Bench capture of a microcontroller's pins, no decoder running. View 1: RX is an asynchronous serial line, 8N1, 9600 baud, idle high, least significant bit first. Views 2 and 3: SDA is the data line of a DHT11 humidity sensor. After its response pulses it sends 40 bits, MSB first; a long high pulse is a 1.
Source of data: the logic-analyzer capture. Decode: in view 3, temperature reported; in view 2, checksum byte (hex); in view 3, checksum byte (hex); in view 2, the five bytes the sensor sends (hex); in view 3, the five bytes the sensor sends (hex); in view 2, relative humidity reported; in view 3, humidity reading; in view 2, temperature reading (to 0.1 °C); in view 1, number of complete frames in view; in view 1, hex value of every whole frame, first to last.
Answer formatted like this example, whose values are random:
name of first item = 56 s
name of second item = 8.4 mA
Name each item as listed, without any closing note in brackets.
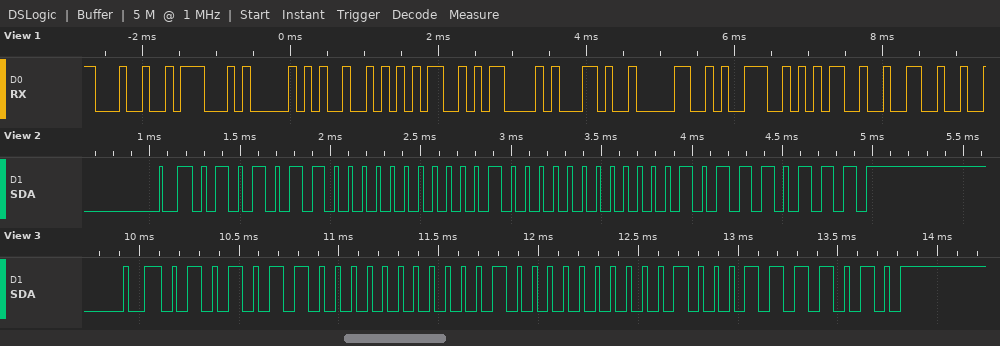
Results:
in view 3, temperature reported = 32.4 °C
in view 2, checksum byte = 0x77
in view 3, checksum byte = 0x7A
in view 2, the five bytes the sensor sends = 56 00 20 01 77
in view 3, the five bytes the sensor sends = 56 00 20 04 7A
in view 2, relative humidity reported = 86 %
in view 3, humidity reading = 86 %
in view 2, temperature reading = 32.1 °C
in view 1, number of complete frames in view = 11
in view 1, hex value of every whole frame, first to last = 0x24 0x47 0x50 0x52 0x4D 0x43 0x2C 0x30 0x39 0x35 0x32
